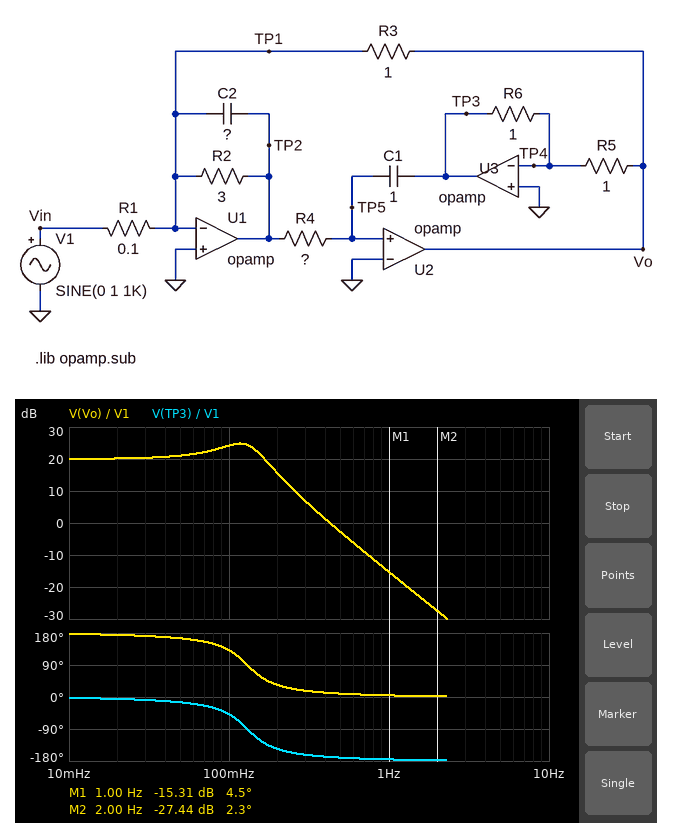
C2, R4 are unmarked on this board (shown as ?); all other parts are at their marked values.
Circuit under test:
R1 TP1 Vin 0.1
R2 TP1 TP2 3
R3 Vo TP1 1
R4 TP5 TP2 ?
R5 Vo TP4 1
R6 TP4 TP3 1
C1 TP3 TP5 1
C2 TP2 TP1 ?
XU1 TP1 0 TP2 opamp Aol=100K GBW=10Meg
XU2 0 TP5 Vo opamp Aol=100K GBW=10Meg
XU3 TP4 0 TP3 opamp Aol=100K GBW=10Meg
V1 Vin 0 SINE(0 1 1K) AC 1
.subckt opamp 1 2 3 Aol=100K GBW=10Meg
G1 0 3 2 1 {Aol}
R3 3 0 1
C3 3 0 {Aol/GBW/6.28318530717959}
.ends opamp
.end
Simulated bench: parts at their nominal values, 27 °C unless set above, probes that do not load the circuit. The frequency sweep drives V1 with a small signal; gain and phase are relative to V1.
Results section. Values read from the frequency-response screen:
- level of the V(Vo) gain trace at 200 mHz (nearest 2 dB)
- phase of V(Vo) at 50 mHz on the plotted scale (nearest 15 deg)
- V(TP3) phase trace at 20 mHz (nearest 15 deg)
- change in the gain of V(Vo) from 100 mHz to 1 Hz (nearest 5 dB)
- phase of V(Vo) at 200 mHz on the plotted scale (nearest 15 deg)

16 dB
165 deg
0 deg
-40 dB
30 deg
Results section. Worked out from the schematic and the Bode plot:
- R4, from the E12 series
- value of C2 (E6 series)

2.2 Ω
680 mF
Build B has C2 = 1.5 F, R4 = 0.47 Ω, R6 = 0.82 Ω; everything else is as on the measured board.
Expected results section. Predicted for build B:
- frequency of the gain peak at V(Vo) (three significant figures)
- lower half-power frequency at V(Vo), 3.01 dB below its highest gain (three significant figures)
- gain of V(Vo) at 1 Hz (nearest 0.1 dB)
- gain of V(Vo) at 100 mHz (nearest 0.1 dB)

208 mHz
189 mHz
-6.8 dB
22.2 dB
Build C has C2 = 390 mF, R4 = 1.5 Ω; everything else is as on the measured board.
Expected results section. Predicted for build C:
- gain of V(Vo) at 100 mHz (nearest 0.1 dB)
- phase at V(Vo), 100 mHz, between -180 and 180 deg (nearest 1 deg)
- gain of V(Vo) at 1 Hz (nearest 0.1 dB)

21.6 dB
158 deg
-7.0 dB
